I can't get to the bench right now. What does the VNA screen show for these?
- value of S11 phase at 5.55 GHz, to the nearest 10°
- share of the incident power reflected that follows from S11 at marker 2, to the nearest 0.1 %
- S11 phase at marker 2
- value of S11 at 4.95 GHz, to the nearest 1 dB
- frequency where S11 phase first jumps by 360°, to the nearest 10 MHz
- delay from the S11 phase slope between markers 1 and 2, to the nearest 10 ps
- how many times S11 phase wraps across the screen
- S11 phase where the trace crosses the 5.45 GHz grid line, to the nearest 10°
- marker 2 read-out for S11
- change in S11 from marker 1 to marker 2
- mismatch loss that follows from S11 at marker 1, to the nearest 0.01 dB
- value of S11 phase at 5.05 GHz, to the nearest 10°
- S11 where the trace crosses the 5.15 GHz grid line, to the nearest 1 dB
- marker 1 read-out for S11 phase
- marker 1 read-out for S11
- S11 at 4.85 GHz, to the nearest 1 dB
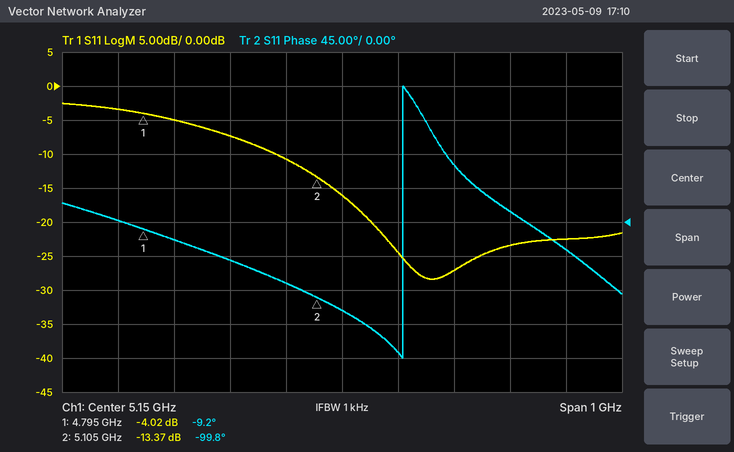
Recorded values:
-40°
4.6 %
-99.8°
-7 dB
5.26 GHz
810 ps
1
10°
-13.37 dB
-9.35 dB
2.19 dB
-80°
-16 dB
-9.2°
-4.02 dB
-5 dB
